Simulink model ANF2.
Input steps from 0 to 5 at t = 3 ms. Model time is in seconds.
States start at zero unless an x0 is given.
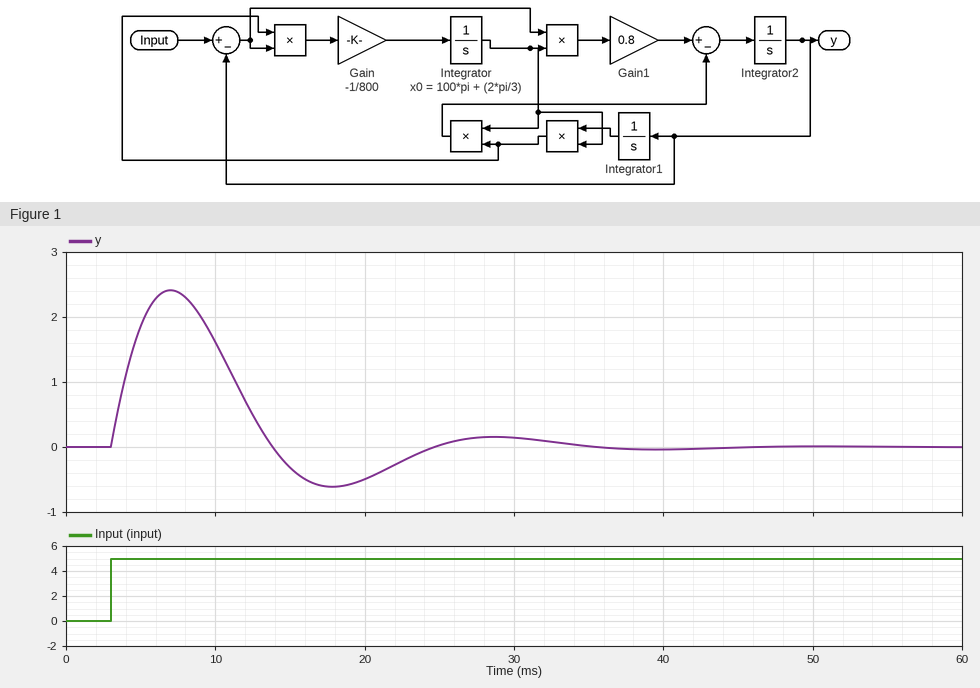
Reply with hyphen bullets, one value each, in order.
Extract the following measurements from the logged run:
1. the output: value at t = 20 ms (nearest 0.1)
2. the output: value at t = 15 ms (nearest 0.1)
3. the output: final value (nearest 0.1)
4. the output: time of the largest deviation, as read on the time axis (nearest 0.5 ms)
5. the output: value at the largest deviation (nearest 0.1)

- -0.5
- -0.3
- 0.0
- 7.0 ms
- 2.4
